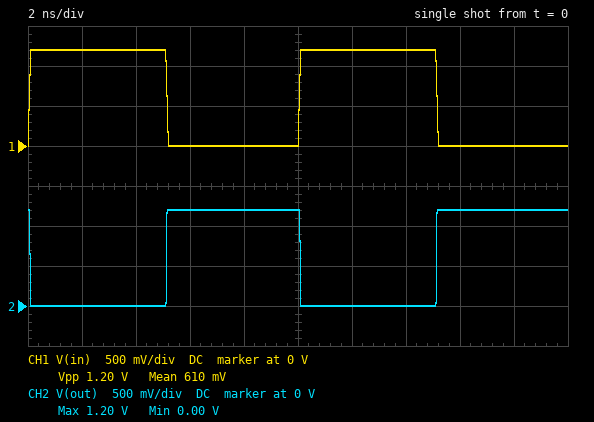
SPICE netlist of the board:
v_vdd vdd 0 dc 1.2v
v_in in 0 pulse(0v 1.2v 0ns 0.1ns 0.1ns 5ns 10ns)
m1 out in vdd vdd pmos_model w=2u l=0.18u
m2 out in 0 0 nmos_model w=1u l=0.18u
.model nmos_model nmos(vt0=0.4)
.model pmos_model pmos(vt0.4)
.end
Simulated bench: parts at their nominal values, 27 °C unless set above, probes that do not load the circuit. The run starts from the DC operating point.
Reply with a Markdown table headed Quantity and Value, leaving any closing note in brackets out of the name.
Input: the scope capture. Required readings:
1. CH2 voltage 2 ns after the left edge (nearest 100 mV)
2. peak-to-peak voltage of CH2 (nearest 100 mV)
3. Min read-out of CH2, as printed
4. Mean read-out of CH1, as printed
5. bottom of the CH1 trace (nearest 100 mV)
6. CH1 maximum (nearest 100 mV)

| Quantity | Value |
|---|---|
| CH2 voltage 2 ns after the left edge | 0 V |
| peak-to-peak voltage of CH2 | 1.2 V |
| Min read-out of CH2, as printed | 0.00 V |
| Mean read-out of CH1, as printed | 610 mV |
| bottom of the CH1 trace | 0 V |
| CH1 maximum | 1.2 V |
